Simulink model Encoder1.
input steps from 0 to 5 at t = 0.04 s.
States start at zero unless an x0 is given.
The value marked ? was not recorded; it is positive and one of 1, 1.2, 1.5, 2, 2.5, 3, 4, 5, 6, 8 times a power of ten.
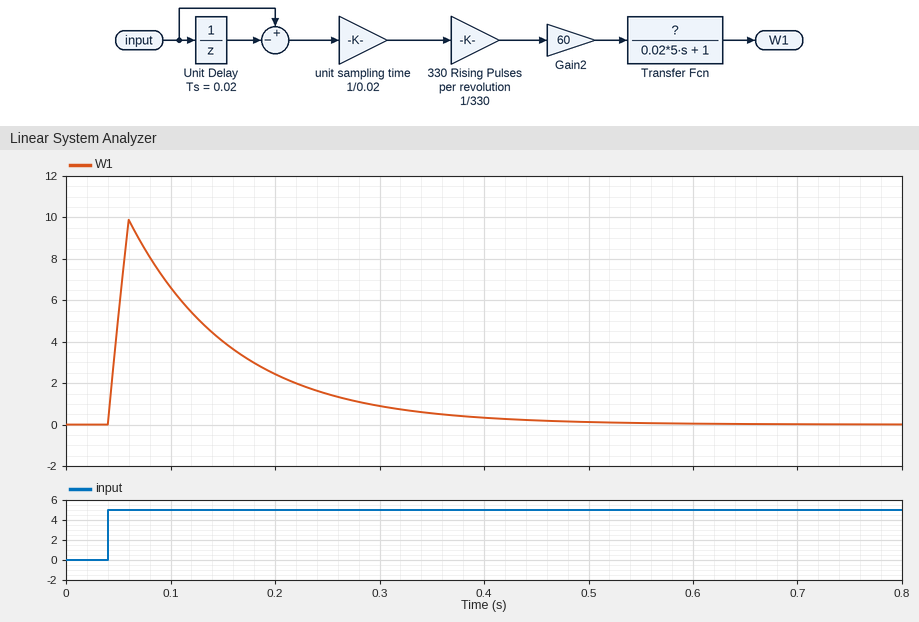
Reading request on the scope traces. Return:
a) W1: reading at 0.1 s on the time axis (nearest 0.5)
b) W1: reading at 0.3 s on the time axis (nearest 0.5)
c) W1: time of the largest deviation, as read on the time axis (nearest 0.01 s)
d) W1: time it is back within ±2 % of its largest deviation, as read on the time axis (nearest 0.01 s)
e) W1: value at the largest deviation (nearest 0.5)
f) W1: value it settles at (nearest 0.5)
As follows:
6.5
1.0
0.06 s
0.45 s
10.0
0.0
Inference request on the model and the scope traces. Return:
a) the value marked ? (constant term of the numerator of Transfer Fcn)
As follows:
1.2
